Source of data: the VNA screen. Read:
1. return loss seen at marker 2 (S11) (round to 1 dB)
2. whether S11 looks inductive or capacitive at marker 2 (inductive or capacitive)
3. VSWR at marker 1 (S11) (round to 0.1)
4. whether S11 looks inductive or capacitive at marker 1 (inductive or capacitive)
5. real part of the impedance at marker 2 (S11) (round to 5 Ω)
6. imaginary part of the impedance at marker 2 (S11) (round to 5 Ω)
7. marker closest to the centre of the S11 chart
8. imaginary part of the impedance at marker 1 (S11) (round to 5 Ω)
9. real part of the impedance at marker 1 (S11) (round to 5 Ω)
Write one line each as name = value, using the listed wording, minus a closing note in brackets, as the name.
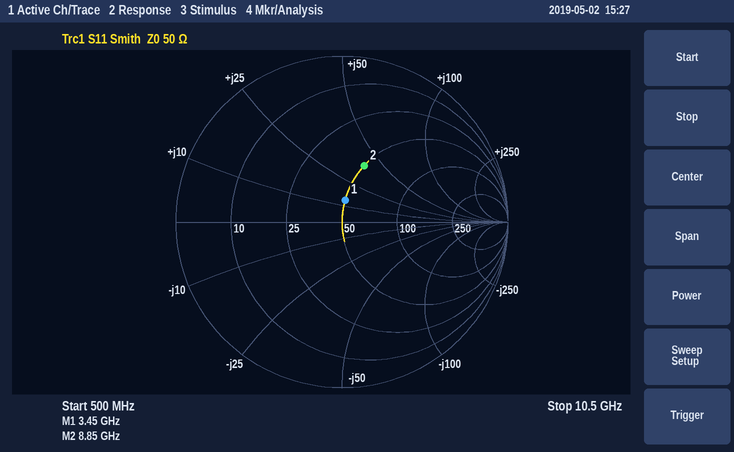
return loss seen at marker 2 (S11) = 9 dB
whether S11 looks inductive or capacitive at marker 2 = inductive
VSWR at marker 1 (S11) = 1.3
whether S11 looks inductive or capacitive at marker 1 = inductive
real part of the impedance at marker 2 (S11) = 50 Ω
imaginary part of the impedance at marker 2 (S11) = +40 Ω
marker closest to the centre of the S11 chart = marker 1
imaginary part of the impedance at marker 1 (S11) = +15 Ω
real part of the impedance at marker 1 (S11) = 50 Ω
